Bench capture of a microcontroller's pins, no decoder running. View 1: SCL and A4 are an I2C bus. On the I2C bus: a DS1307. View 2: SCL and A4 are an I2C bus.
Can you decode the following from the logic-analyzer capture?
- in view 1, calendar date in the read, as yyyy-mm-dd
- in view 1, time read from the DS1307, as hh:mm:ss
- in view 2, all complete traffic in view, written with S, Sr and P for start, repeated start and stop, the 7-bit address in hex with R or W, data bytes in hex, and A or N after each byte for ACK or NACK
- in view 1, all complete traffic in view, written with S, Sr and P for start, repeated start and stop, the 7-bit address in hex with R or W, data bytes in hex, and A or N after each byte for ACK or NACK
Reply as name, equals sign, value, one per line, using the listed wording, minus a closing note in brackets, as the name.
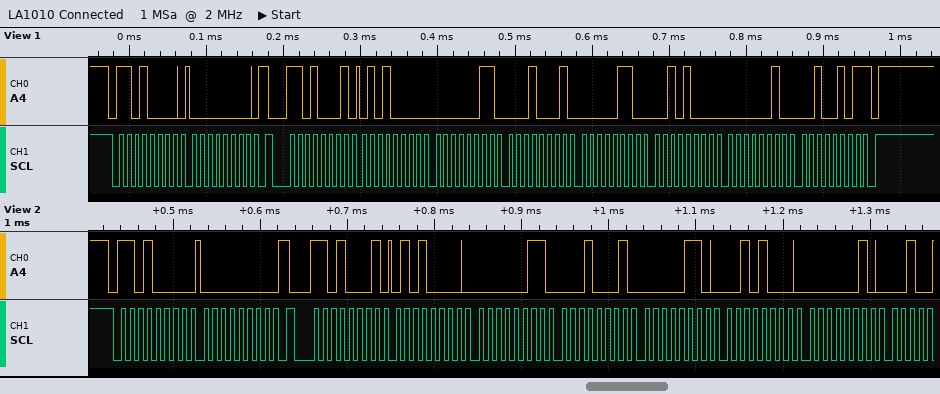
in view 1, calendar date in the read, as yyyy-mm-dd = 2025-02-28
in view 1, time read from the DS1307, as hh:mm:ss = 11:03:50
in view 2, all complete traffic in view, written with S, Sr and P for start, repeated start and stop, the 7-bit address in hex with R or W, data bytes in hex, and A or N after each byte for ACK or NACK = S 68W A 00 A Sr 68R A 50 A 03 A 11 A 06 A 28 A 02 A
in view 1, all complete traffic in view, written with S, Sr and P for start, repeated start and stop, the 7-bit address in hex with R or W, data bytes in hex, and A or N after each byte for ACK or NACK = S 68W A 00 A Sr 68R A 50 A 03 A 11 A 06 A 28 A 02 A 25 N P
